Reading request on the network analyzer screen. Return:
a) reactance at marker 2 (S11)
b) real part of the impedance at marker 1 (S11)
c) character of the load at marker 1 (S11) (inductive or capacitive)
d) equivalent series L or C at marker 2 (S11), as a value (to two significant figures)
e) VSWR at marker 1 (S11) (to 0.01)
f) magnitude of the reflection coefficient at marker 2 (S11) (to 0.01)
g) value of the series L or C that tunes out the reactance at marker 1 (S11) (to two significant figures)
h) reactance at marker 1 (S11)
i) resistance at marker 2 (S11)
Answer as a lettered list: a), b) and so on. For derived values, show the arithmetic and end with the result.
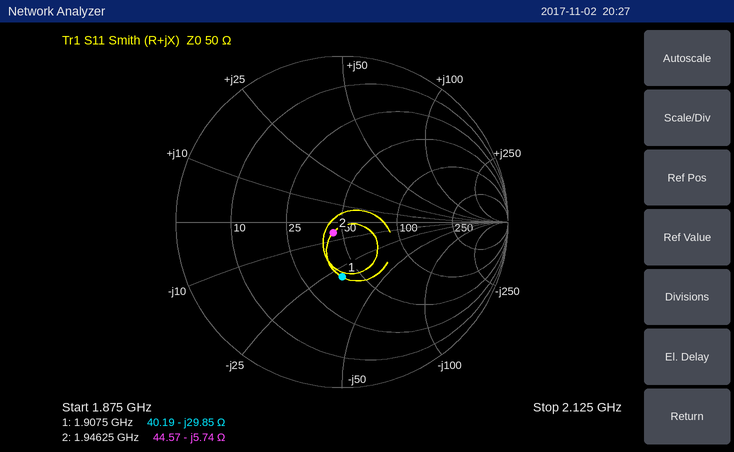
a) -5.74 Ω
b) 40.19 Ω
c) capacitive
d) C = 1/(2π × 1.94625 GHz × 5.74 Ω) ≈ 14 pF
e) 1.99
f) 0.08
g) L = 29.85 Ω/(2π × 1.9075 GHz) ≈ 2.5 nH
h) -29.85 Ω
i) 44.57 Ω
